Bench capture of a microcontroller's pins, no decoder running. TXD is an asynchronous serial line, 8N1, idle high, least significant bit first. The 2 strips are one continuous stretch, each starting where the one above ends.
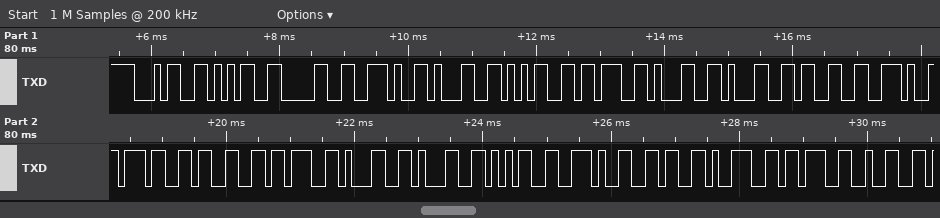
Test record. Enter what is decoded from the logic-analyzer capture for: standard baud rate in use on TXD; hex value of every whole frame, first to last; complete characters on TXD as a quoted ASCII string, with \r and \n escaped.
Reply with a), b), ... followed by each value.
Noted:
a) 9600 baud
b) 34 35 30 2E 31 35 3B 31 31 33 2E 37 33 3B 31 31 35 2E 36 39 3B 32
c) "450.15;113.73;115.69;2"
